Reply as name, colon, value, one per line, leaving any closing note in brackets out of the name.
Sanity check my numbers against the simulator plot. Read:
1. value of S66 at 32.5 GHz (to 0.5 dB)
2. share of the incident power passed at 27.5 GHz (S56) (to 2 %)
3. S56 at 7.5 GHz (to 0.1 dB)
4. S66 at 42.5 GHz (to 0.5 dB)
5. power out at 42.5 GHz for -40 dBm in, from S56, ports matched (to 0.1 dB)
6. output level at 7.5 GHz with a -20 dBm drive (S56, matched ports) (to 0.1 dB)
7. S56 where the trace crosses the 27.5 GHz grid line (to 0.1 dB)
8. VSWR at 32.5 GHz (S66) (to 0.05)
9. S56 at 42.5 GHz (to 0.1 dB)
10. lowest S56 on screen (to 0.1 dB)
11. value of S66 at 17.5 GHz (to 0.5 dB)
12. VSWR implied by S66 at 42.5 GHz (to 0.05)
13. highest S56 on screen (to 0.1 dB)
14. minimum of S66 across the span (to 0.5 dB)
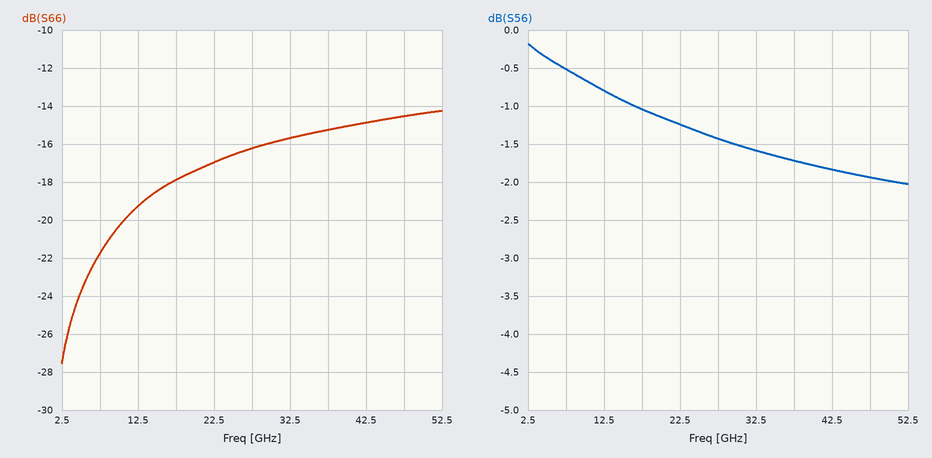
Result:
value of S66 at 32.5 GHz: -15.5 dB
share of the incident power passed at 27.5 GHz (S56): 72 %
S56 at 7.5 GHz: -0.5 dB
S66 at 42.5 GHz: -15.0 dB
power out at 42.5 GHz for -40 dBm in, from S56, ports matched: -41.8 dBm
output level at 7.5 GHz with a -20 dBm drive (S56, matched ports): -20.5 dBm
S56 where the trace crosses the 27.5 GHz grid line: -1.4 dB
VSWR at 32.5 GHz (S66): 1.40
S56 at 42.5 GHz: -1.8 dB
lowest S56 on screen: -2.0 dB
value of S66 at 17.5 GHz: -18.0 dB
VSWR implied by S66 at 42.5 GHz: 1.45
highest S56 on screen: -0.2 dB
minimum of S66 across the span: -27.5 dB
